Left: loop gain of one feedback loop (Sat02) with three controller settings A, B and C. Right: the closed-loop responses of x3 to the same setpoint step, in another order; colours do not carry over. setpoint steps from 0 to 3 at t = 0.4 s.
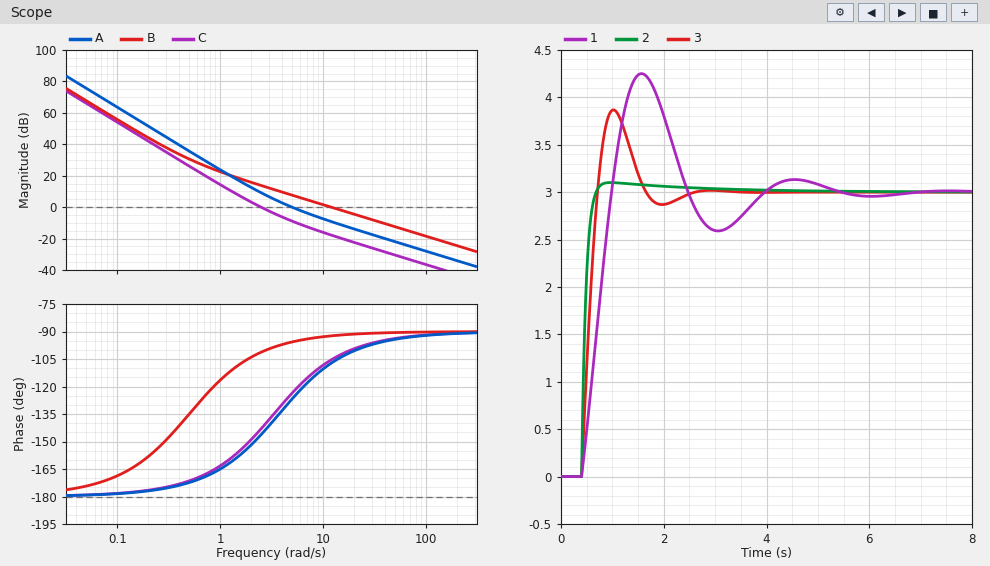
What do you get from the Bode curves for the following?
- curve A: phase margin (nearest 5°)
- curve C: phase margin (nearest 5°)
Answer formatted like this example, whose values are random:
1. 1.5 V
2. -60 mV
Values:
1. 55°
2. 35°
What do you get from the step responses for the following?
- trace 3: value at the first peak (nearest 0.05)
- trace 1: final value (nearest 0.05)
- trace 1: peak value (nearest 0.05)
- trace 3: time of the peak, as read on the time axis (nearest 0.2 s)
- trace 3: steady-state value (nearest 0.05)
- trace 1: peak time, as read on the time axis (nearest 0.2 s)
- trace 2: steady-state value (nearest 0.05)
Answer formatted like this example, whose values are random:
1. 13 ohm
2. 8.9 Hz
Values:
1. 3.85
2. 3.00
3. 4.25
4. 1.0 s
5. 3.00
6. 1.6 s
7. 3.00
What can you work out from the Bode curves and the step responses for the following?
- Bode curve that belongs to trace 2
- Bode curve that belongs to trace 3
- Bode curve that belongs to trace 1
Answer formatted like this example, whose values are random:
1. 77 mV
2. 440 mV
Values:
1. B
2. A
3. C
